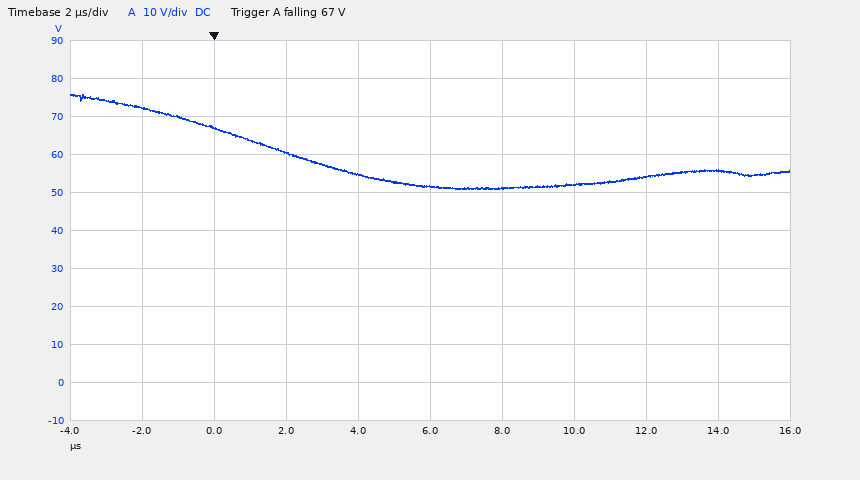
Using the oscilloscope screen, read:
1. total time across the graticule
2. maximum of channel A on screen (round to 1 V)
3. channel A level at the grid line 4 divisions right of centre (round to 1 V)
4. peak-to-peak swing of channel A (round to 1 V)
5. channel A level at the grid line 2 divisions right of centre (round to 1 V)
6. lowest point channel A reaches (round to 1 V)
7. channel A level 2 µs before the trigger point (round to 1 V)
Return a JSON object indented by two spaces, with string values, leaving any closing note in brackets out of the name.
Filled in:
{
  "total time across the graticule": "20 µs",
  "maximum of channel A on screen": "76 V",
  "channel A level at the grid line 4 divisions right of centre": "56 V",
  "peak-to-peak swing of channel A": "25 V",
  "channel A level at the grid line 2 divisions right of centre": "52 V",
  "lowest point channel A reaches": "51 V",
  "channel A level 2 µs before the trigger point": "72 V"
}
